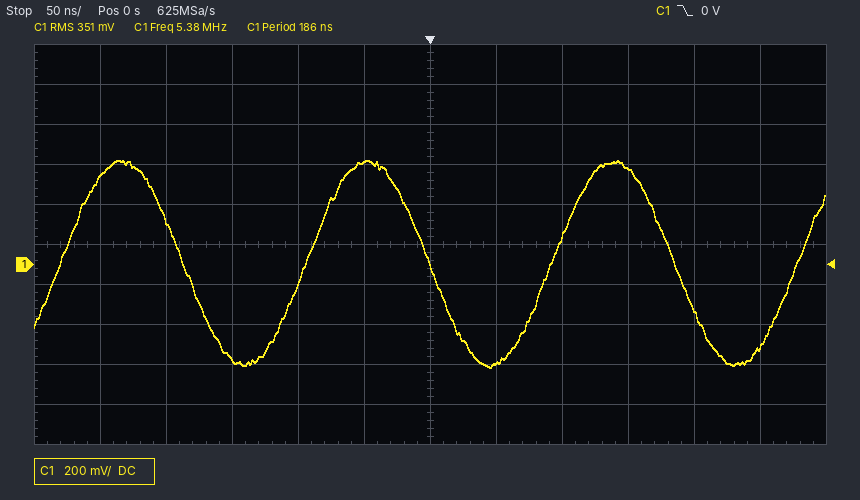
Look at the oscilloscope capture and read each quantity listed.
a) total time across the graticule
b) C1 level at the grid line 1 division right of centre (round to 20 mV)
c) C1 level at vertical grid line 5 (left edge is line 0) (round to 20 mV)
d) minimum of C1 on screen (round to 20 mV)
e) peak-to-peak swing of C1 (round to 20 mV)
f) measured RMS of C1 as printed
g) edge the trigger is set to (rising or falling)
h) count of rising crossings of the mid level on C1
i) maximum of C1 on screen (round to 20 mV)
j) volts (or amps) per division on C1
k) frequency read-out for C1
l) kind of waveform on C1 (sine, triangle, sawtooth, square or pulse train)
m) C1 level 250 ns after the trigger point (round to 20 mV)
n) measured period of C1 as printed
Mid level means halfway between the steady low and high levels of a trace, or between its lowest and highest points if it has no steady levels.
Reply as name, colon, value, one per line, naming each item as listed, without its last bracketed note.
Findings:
total time across the graticule: 600 ns
C1 level at the grid line 1 division right of centre: -500 mV
C1 level at vertical grid line 5 (left edge is line 0): 520 mV
minimum of C1 on screen: -520 mV
peak-to-peak swing of C1: 1.04 V
measured RMS of C1 as printed: 351 mV
edge the trigger is set to: falling
count of rising crossings of the mid level on C1: 4
maximum of C1 on screen: 520 mV
volts (or amps) per division on C1: 200 mV
frequency read-out for C1: 5.38 MHz
kind of waveform on C1: sine
C1 level 250 ns after the trigger point: -420 mV
measured period of C1 as printed: 186 ns
